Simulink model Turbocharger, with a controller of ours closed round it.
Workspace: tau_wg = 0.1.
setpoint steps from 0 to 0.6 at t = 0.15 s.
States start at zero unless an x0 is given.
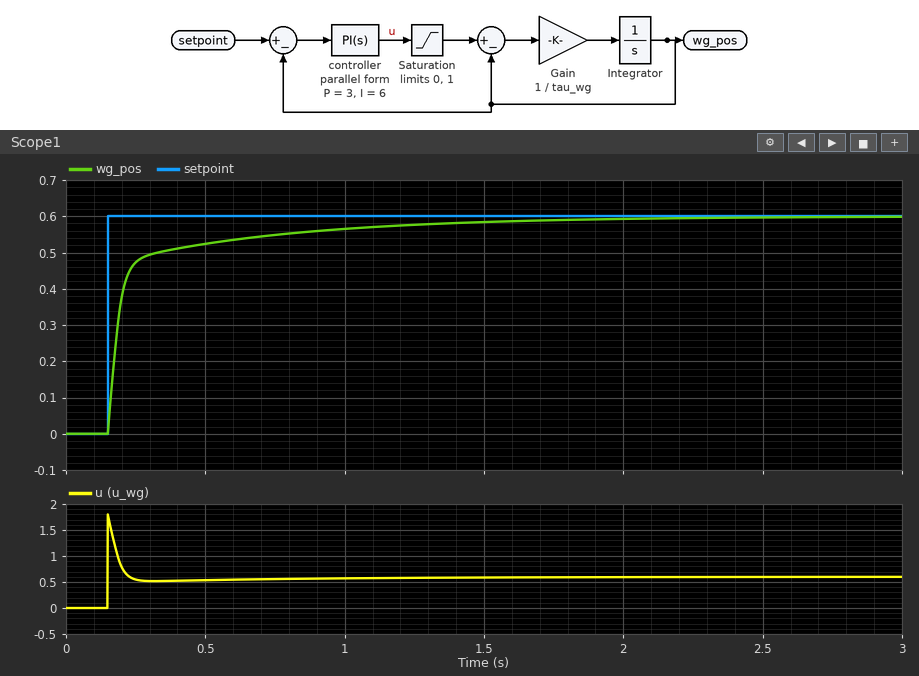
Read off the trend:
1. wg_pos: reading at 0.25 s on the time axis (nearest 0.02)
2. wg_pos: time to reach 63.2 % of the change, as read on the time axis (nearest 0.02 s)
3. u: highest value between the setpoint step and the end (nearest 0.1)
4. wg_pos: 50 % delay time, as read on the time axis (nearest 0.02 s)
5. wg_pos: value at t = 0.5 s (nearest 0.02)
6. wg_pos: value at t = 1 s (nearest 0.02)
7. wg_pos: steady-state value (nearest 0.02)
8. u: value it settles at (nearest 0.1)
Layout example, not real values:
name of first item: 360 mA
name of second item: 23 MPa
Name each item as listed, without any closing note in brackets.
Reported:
wg_pos: reading at 0.25 s on the time axis: 0.48
wg_pos: time to reach 63.2 % of the change, as read on the time axis: 0.20 s
u: highest value between the setpoint step and the end: 1.8
wg_pos: 50 % delay time, as read on the time axis: 0.18 s
wg_pos: value at t = 0.5 s: 0.52
wg_pos: value at t = 1 s: 0.56
wg_pos: steady-state value: 0.60
u: value it settles at: 0.6
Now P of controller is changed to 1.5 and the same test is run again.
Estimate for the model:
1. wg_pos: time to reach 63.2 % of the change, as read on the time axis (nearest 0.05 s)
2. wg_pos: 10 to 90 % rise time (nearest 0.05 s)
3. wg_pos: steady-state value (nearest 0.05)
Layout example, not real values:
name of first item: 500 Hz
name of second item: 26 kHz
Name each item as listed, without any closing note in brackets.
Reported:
wg_pos: time to reach 63.2 % of the change, as read on the time axis: 0.25 s
wg_pos: 10 to 90 % rise time: 0.50 s
wg_pos: steady-state value: 0.60
